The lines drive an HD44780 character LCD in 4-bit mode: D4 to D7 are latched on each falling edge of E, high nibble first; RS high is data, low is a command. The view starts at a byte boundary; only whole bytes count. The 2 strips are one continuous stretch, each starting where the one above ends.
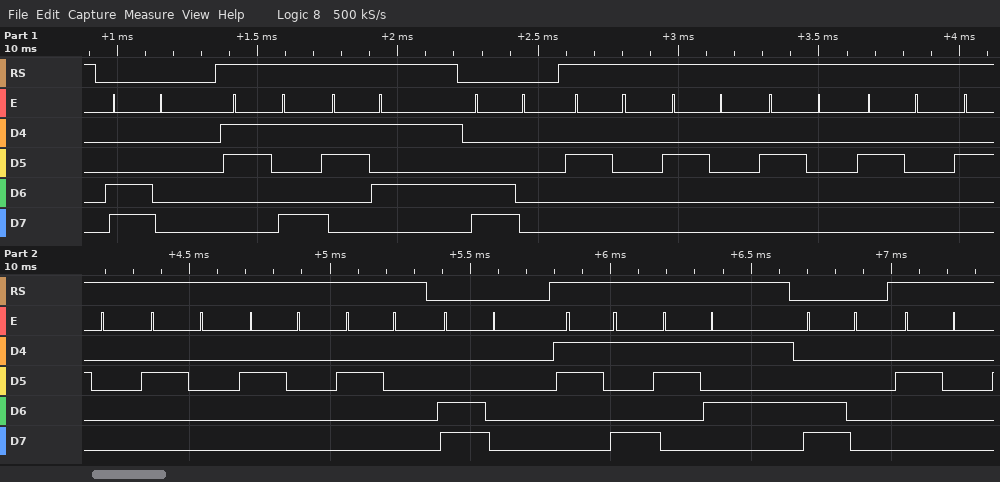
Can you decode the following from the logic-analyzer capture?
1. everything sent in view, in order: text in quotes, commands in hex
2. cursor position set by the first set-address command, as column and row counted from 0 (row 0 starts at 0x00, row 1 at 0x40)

0xC0 "95" 0xC0 "        " 0xC0 "95" 0xC0 " "
column 0, row 1
